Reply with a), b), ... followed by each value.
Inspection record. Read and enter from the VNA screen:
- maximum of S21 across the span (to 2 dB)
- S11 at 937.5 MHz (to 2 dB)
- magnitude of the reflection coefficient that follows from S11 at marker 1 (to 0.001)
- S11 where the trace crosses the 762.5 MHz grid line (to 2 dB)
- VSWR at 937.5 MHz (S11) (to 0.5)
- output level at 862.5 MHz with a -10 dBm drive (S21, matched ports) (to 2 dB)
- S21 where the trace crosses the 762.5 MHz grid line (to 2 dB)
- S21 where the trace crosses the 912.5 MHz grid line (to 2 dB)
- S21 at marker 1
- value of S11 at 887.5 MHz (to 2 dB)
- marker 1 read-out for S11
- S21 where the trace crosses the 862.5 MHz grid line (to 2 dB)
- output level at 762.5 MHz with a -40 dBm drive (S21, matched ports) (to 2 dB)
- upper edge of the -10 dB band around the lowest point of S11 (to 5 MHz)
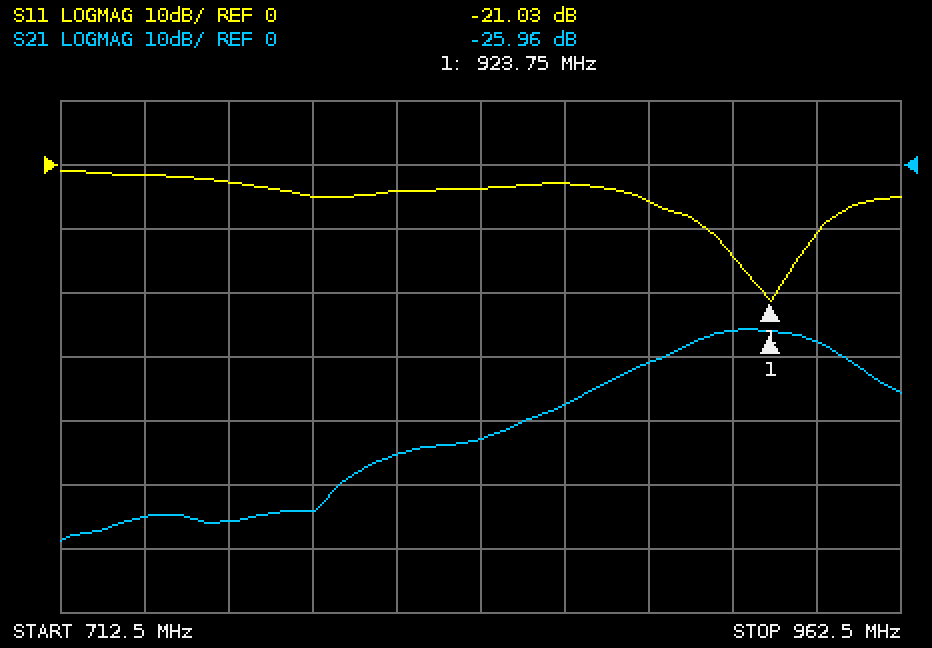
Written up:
a) -26 dB
b) -10 dB
c) 0.089
d) -2 dB
e) 2.0
f) -48 dBm
g) -56 dB
h) -26 dB
i) -25.96 dB
j) -6 dB
k) -21.03 dB
l) -38 dB
m) -96 dBm
n) 940 MHz
